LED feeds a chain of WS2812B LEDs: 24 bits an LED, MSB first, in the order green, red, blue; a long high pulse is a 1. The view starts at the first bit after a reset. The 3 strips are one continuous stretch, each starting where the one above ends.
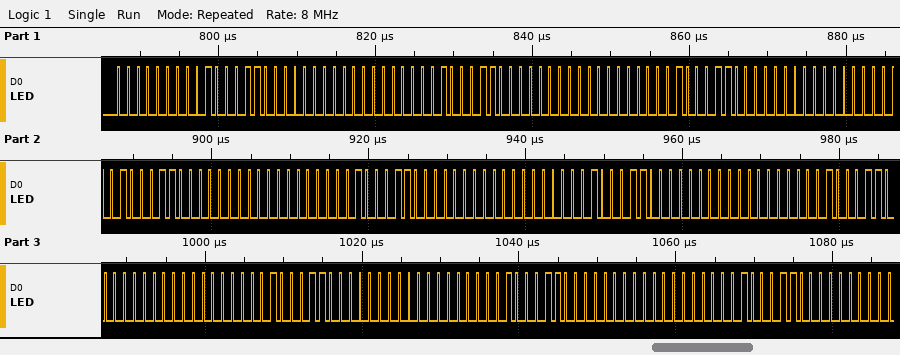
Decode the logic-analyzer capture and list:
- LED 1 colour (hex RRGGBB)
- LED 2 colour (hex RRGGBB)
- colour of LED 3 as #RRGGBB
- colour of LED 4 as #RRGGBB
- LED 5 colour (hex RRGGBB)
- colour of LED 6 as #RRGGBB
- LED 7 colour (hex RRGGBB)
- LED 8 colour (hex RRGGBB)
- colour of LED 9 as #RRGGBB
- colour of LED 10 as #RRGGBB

#460000
#460000
#460000
#460000
#460000
#460000
#460000
#460000
#460000
#460000
